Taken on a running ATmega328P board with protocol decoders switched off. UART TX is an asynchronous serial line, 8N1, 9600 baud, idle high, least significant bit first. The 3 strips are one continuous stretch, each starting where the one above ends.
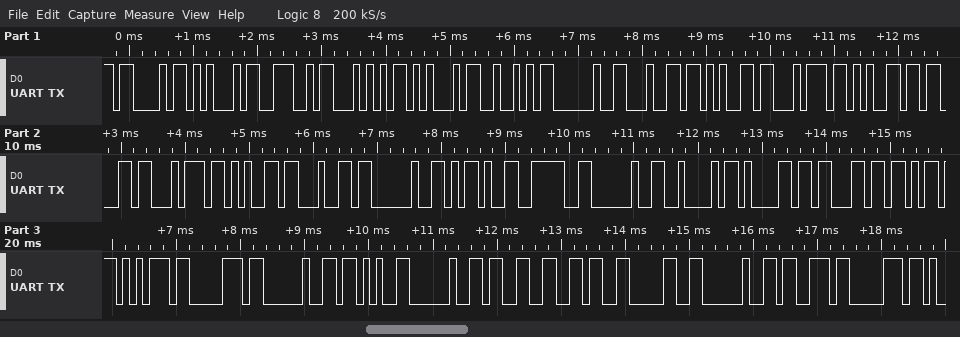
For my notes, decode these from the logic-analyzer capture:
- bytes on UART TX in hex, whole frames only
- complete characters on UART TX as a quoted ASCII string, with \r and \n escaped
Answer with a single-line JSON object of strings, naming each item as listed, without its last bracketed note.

{"bytes on UART TX in hex, whole frames only": "43 45 4E 54 45 52 20 64 65 74 65 63 74 65 64 20 2D 3E 20 42 61 63 6B 75 70 20 2B 20 33 36 30 20 73 70", "complete characters on UART TX as a quoted ASCII string, with \\r and \\n escaped": "\"CENTER detected -> Backup + 360 sp\""}
